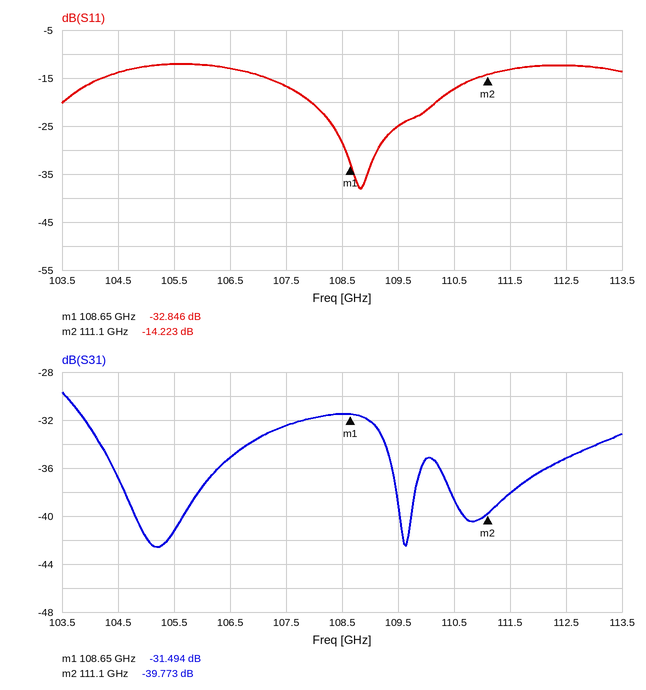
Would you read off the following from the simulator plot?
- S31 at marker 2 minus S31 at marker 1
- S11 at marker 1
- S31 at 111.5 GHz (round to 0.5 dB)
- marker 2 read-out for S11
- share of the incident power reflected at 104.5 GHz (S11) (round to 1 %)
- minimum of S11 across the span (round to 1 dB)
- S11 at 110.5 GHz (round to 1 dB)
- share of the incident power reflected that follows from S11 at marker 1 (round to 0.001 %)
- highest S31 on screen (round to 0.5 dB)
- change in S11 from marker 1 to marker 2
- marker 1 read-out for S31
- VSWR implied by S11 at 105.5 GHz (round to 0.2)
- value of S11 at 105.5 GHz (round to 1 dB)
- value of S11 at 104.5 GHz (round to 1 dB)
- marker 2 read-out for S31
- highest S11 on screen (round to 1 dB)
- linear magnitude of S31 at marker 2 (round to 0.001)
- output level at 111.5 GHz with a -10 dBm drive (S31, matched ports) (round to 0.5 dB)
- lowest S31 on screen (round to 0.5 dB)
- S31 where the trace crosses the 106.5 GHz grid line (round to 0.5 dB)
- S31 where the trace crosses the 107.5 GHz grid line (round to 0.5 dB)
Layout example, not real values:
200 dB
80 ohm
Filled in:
-8.279 dB
-32.846 dB
-38.0 dB
-14.223 dB
4 %
-38 dB
-17 dB
0.052 %
-29.5 dB
18.623 dB
-31.494 dB
1.6
-12 dB
-14 dB
-39.773 dB
-12 dB
0.010
-48.0 dBm
-42.5 dB
-35.0 dB
-32.5 dB
